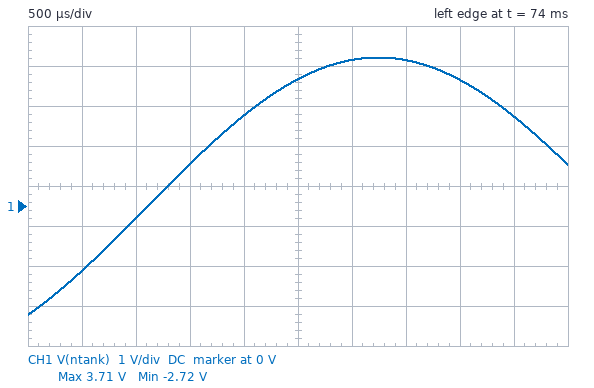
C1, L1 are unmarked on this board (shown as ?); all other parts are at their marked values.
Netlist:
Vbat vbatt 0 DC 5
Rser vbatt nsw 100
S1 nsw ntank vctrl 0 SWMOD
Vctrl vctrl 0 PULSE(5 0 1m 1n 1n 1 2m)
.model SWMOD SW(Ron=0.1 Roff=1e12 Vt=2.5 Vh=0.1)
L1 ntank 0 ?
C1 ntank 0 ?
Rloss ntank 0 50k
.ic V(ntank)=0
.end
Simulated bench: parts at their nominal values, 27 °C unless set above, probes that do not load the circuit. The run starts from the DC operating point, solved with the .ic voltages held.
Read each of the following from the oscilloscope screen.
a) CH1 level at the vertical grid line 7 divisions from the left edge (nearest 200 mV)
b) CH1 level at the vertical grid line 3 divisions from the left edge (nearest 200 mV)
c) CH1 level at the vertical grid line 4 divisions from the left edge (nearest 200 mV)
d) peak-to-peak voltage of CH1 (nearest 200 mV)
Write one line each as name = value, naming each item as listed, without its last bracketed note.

CH1 level at the vertical grid line 7 divisions from the left edge = 3.6 V
CH1 level at the vertical grid line 3 divisions from the left edge = 1.0 V
CH1 level at the vertical grid line 4 divisions from the left edge = 2.2 V
peak-to-peak voltage of CH1 = 6.4 V
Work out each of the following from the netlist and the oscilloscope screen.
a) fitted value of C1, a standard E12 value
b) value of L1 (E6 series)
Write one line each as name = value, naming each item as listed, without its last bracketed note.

fitted value of C1, a standard E12 value = 5.6 µF
value of L1 = 330 mH
